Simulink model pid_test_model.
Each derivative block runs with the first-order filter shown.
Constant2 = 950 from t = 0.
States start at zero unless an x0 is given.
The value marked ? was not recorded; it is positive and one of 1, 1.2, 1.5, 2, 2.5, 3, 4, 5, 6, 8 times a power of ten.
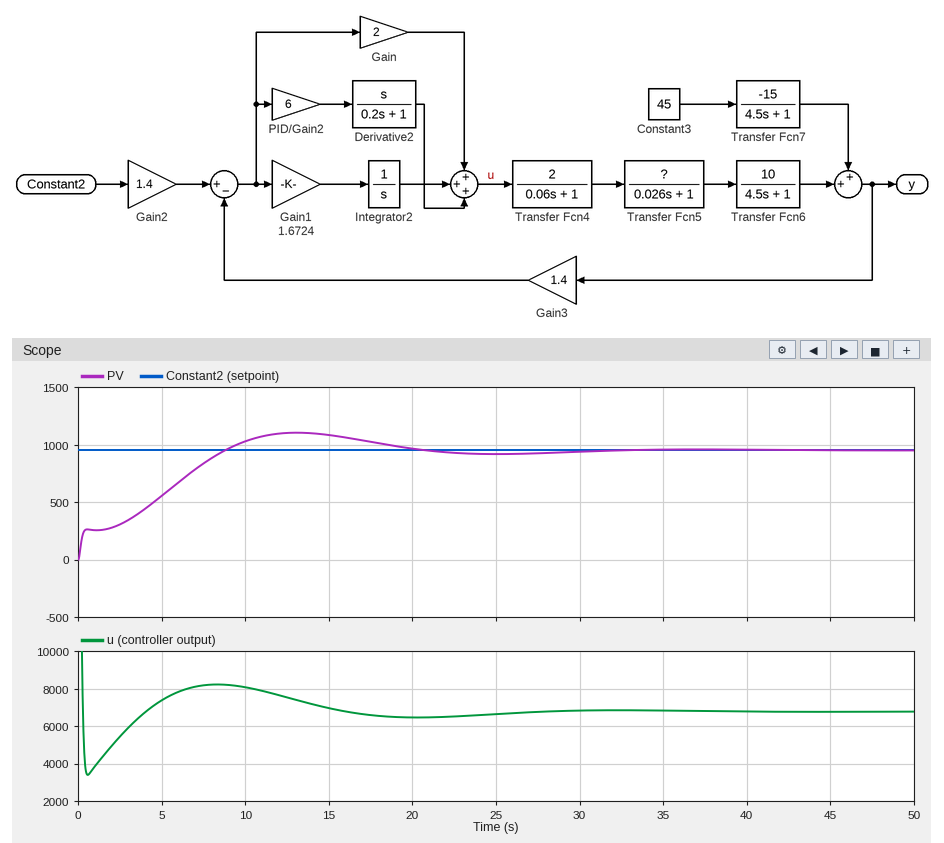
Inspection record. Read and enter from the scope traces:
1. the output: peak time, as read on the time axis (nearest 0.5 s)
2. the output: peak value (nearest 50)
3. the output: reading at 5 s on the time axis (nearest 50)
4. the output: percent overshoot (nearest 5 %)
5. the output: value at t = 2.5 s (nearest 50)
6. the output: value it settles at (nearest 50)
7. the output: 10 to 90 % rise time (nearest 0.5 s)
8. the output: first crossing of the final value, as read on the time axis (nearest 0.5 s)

13.0 s
1100
550
15 %
300
950
7.5 s
9.0 s
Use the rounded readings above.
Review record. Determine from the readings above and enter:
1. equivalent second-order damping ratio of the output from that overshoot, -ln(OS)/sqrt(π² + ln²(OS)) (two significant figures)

0.52
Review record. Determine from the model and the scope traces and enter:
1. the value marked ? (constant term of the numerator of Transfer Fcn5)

0.012
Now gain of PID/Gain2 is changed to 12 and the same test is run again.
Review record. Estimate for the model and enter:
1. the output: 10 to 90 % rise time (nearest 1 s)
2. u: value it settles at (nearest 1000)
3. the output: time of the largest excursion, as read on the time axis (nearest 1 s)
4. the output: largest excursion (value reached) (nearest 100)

9 s
7000
15 s
1100
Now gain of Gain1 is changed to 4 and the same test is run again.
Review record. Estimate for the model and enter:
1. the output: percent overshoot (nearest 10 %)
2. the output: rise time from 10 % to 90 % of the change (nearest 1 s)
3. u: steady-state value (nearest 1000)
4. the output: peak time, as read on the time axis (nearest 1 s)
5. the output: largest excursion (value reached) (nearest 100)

30 %
4 s
7000
8 s
1200
